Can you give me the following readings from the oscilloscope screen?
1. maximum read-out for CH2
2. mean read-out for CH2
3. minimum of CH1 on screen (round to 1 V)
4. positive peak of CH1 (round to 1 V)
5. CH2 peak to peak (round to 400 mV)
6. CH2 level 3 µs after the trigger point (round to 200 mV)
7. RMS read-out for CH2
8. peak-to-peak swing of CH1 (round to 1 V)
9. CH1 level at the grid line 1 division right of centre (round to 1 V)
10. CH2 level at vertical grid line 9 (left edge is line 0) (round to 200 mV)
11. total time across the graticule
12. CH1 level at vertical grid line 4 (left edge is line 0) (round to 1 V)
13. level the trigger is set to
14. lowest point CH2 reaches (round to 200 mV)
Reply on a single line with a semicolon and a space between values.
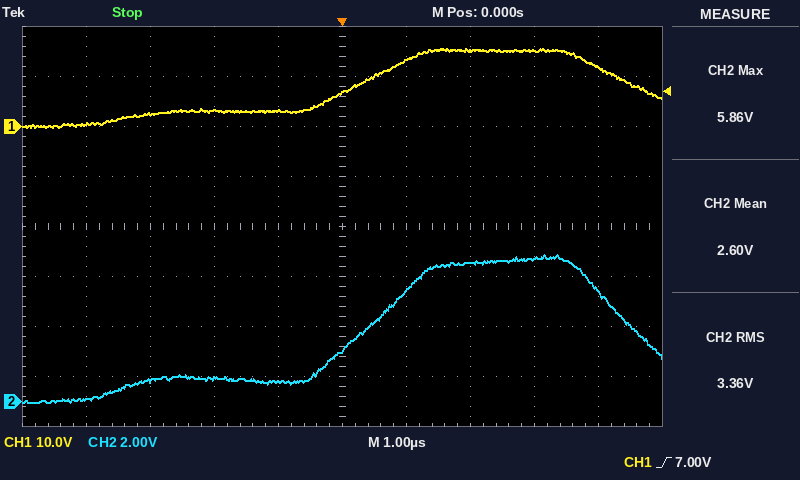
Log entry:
5.86 V; 2.60 V; 0 V; 16 V; 6.0 V; 5.8 V; 3.36 V; 16 V; 13 V; 4.4 V; 10 µs; 3 V; 7.00 V; 0.0 V
